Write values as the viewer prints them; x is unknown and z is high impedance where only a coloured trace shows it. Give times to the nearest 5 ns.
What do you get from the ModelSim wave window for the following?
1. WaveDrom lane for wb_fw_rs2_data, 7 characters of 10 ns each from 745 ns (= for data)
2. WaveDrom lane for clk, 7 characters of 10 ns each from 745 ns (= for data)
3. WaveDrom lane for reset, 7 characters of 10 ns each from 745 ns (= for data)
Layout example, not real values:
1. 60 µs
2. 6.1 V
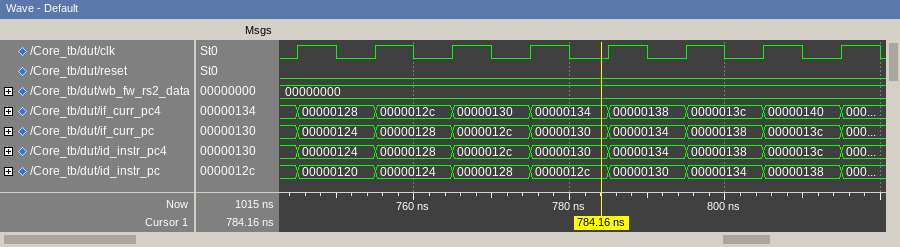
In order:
1. {name: 'wb_fw_rs2_data', wave: '=......', data: '00000000'}
2. {name: 'clk', wave: 'p......'}
3. {name: 'reset', wave: '0......'}
